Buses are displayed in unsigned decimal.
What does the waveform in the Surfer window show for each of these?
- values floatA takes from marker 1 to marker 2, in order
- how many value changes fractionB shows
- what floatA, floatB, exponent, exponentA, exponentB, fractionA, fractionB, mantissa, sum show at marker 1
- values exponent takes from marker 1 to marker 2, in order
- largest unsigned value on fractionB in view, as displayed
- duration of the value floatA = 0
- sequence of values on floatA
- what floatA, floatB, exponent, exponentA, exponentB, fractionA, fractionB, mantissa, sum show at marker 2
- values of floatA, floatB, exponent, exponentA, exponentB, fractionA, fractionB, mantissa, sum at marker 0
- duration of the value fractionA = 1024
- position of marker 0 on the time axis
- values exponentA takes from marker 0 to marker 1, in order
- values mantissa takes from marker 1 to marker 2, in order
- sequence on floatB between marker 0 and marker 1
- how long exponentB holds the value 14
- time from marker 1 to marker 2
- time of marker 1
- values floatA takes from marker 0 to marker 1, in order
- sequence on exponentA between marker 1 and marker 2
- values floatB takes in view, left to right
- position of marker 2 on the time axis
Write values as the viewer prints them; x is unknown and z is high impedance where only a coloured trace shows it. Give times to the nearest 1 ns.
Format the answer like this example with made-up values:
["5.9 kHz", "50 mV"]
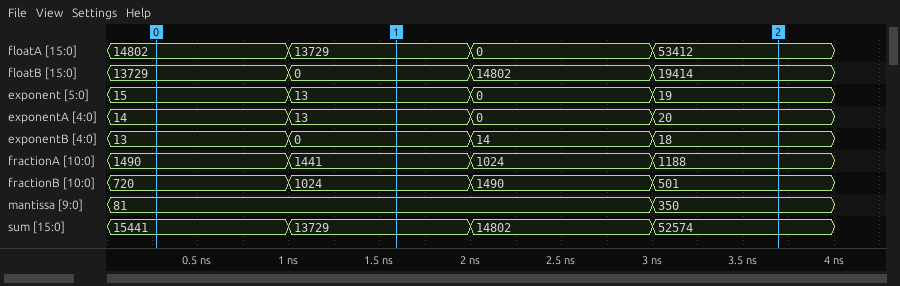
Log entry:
["13729, 0, 53412", "3", "floatA=13729, floatB=0, exponent=13, exponentA=13, exponentB=0, fractionA=1441, fractionB=1024, mantissa=81, sum=13729", "13, 0, 19", "1490", "1 ns", "14802, 13729, 0, 53412", "floatA=53412, floatB=19414, exponent=19, exponentA=20, exponentB=18, fractionA=1188, fractionB=501, mantissa=350, sum=52574", "floatA=14802, floatB=13729, exponent=15, exponentA=14, exponentB=13, fractionA=1490, fractionB=720, mantissa=81, sum=15441", "1 ns", "0 ns", "14, 13", "81, 350", "13729, 0", "1 ns", "2 ns", "2 ns", "14802, 13729", "13, 0, 20", "13729, 0, 14802, 19414", "4 ns"]
